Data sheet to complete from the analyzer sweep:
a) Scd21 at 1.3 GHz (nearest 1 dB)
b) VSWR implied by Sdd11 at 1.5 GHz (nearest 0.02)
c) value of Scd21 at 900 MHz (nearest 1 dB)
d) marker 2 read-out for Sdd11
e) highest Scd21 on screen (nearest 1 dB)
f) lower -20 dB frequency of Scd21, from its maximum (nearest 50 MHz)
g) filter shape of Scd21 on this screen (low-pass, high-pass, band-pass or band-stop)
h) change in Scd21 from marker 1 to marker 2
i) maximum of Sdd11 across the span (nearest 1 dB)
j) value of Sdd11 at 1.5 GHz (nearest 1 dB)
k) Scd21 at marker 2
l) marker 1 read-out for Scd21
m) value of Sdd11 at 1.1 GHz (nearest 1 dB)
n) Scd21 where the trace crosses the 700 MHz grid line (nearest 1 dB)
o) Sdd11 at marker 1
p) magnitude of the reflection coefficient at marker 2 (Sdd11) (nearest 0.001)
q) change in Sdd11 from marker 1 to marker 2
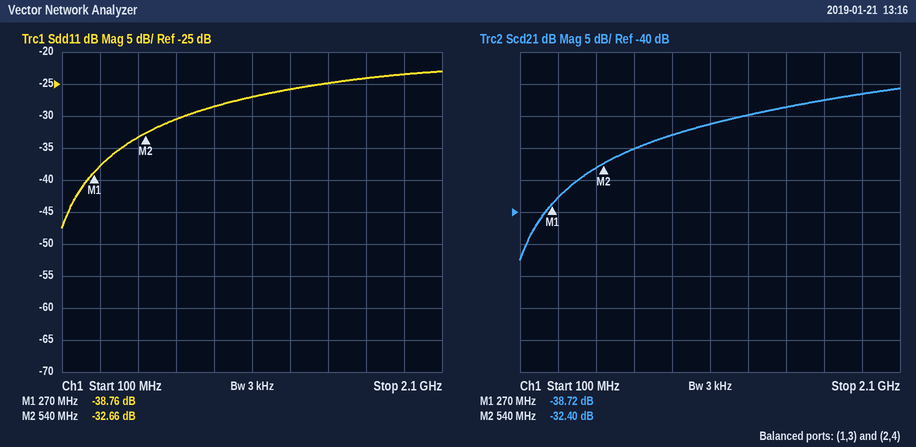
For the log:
-25 dB
1.12
-28 dB
-32.66 dB
-21 dB
200 MHz
high-pass
6.32 dB
-23 dB
-25 dB
-32.40 dB
-38.72 dB
-27 dB
-30 dB
-38.76 dB
0.023
6.10 dB
